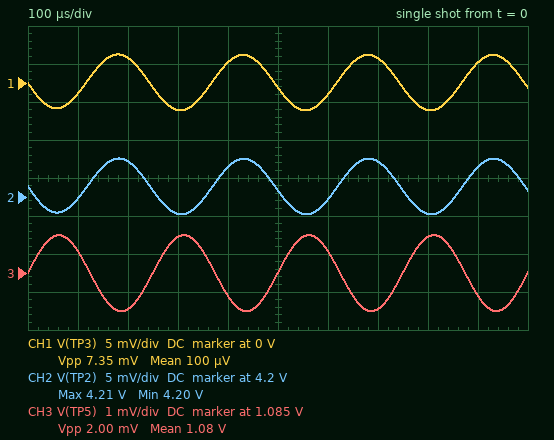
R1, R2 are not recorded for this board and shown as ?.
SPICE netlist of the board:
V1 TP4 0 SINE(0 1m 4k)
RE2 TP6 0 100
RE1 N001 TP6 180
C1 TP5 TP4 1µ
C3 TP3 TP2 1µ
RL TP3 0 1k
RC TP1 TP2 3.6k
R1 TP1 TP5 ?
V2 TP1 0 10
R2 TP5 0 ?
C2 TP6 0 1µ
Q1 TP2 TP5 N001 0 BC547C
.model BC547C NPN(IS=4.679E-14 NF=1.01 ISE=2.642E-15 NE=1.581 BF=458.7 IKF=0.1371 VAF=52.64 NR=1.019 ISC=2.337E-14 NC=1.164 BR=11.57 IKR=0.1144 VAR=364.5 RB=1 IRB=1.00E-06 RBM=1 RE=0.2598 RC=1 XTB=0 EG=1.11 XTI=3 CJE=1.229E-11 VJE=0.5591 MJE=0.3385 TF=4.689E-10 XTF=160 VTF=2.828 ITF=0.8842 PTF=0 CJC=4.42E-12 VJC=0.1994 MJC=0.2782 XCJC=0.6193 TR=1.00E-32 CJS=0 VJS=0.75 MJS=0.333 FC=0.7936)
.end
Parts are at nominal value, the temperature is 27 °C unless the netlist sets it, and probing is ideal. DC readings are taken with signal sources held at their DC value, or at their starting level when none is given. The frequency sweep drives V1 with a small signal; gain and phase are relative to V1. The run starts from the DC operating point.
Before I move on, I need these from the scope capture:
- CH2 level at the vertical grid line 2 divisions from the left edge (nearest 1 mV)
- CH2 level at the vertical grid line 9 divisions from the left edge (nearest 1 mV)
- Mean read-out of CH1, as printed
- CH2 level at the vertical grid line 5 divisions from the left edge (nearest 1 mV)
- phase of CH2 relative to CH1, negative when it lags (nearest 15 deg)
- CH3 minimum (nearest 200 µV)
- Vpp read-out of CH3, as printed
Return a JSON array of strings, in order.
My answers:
["4.205 V", "4.204 V", "100 µV", "4.201 V", "0 deg", "1.0840 V", "2.00 mV"]
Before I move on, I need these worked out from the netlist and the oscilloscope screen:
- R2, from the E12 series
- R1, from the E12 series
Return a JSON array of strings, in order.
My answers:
["2.7 kΩ", "22 kΩ"]
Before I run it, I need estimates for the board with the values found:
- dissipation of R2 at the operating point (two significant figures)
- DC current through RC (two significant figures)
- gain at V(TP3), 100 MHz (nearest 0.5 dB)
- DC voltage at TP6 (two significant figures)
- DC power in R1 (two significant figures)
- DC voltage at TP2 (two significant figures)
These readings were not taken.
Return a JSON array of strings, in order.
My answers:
["440 µW", "1.6 mA", "9.0 dB", "160 mV", "3.6 mW", "4.2 V"]
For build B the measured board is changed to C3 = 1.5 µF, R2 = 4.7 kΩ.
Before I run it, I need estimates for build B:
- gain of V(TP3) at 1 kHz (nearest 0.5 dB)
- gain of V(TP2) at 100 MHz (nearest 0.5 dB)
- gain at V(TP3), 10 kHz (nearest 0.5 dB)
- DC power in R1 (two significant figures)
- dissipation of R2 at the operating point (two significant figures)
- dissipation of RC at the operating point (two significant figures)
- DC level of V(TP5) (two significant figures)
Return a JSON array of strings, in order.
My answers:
["-20.5 dB", "0 dB", "-16.0 dB", "3.4 mW", "420 µW", "24 mW", "1.4 V"]
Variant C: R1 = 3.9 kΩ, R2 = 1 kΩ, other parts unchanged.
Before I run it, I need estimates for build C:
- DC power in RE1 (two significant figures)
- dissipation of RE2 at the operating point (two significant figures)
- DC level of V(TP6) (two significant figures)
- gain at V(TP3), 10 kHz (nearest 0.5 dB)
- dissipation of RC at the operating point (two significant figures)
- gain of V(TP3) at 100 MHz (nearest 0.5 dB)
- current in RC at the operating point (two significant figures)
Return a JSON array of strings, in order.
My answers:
["1.8 mW", "980 µW", "310 mV", "-2.5 dB", "23 mW", "0 dB", "2.5 mA"]
